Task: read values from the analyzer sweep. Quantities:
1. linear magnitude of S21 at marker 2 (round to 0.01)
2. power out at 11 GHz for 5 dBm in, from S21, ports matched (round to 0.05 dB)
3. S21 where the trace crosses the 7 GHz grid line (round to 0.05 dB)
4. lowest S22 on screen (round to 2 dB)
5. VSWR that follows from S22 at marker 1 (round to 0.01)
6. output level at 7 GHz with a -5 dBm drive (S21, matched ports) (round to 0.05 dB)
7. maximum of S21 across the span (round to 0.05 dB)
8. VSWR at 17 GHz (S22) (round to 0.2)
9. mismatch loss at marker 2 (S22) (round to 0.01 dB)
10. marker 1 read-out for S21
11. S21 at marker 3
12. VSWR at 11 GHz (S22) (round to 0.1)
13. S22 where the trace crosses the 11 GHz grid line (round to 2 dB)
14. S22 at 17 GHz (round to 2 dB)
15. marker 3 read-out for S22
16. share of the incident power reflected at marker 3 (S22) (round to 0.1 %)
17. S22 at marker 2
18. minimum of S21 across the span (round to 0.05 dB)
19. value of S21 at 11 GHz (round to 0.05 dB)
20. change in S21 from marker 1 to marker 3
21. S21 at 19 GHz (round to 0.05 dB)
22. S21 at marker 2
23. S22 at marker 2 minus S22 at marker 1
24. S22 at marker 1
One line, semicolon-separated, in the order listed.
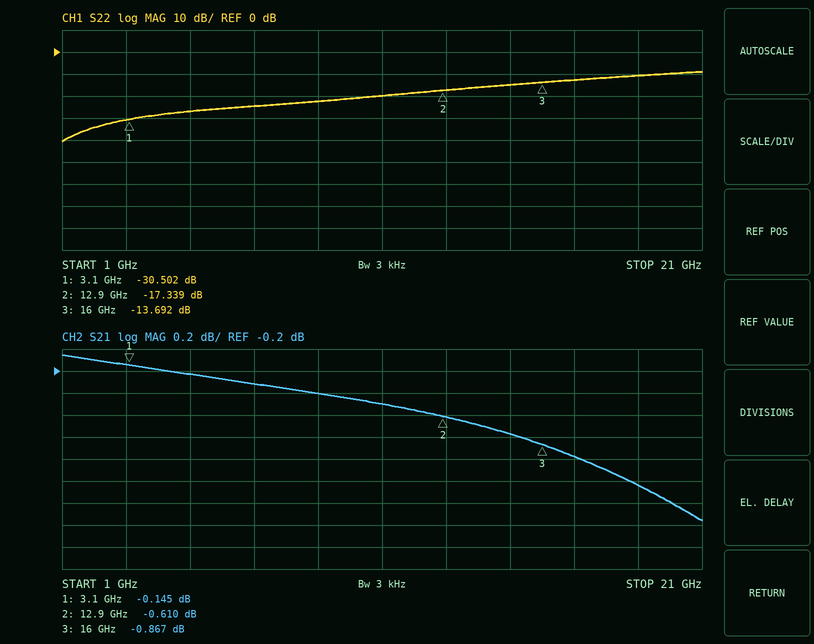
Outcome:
0.93; 4.50 dBm; -0.30 dB; -40 dB; 1.06; -5.30 dBm; -0.05 dB; 1.6; 0.08 dB; -0.145 dB; -0.867 dB; 1.2; -20 dB; -12 dB; -13.692 dB; 4.3 %; -17.339 dB; -1.55 dB; -0.50 dB; -0.722 dB; -1.25 dB; -0.610 dB; 13.163 dB; -30.502 dB
